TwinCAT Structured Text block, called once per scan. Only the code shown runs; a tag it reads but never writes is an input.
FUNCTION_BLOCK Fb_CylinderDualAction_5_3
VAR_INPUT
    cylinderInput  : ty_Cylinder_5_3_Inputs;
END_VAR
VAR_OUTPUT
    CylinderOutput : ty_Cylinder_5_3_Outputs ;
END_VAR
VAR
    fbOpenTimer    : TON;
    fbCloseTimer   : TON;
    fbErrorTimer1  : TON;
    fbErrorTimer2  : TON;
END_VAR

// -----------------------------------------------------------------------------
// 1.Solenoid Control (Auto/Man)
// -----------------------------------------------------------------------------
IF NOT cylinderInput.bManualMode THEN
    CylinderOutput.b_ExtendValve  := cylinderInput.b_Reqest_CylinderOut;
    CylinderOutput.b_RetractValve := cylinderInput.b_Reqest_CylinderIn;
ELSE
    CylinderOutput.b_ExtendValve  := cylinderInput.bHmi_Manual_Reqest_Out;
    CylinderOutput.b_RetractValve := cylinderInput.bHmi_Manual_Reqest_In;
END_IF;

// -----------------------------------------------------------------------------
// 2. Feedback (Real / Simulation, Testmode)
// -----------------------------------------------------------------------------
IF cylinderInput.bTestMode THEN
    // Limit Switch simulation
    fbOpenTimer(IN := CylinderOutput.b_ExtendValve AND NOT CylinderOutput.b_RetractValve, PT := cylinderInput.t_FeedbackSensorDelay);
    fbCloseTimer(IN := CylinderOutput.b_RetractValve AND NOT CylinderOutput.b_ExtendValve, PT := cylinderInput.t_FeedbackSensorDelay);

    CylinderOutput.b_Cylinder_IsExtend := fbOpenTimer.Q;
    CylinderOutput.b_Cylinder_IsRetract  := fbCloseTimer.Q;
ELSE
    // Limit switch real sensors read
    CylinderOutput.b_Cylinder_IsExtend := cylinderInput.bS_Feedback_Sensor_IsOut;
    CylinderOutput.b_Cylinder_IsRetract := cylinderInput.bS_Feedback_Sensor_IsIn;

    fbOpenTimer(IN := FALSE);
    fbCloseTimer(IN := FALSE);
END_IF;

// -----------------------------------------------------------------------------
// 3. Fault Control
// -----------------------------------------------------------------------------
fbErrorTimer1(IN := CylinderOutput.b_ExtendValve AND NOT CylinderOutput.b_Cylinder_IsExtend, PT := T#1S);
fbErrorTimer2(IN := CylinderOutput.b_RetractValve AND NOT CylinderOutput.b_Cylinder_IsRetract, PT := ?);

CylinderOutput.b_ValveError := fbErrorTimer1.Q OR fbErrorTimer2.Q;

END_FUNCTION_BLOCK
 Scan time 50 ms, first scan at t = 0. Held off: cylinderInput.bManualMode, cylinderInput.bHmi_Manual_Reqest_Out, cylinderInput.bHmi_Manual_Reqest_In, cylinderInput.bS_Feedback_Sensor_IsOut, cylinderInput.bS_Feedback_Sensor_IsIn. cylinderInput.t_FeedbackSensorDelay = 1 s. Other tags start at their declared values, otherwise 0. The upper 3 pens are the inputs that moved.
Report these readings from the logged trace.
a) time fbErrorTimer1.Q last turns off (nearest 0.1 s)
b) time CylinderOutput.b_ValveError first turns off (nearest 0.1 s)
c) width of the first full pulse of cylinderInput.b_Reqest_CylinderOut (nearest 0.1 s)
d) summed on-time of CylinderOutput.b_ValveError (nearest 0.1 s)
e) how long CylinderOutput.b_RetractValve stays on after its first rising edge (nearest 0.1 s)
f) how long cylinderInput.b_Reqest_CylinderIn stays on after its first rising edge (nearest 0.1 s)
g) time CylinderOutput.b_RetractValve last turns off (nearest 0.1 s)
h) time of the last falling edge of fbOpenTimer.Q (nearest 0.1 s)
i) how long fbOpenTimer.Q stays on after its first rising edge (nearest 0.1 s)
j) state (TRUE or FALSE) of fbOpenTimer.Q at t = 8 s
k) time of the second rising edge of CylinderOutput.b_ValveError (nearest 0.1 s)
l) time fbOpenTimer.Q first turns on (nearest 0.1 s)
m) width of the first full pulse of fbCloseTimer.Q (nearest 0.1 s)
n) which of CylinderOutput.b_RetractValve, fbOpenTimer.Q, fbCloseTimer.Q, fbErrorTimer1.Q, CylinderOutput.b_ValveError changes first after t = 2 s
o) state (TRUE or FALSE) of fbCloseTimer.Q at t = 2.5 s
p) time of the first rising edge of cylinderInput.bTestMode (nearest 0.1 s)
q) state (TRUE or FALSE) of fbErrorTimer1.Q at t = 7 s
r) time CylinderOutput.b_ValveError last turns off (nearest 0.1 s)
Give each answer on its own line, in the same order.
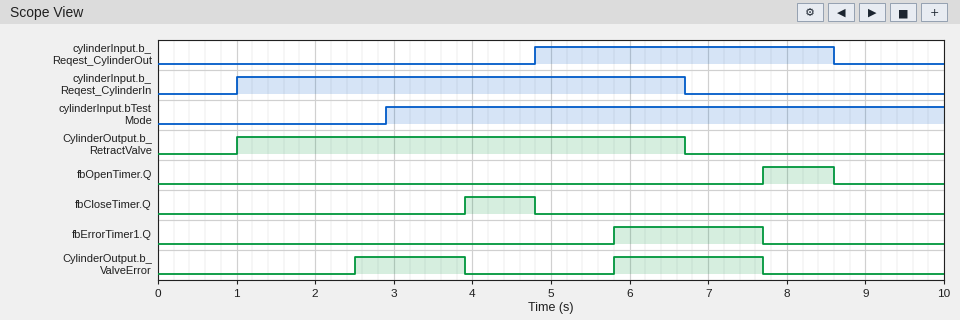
7.7 s
3.9 s
3.8 s
3.3 s
5.7 s
5.7 s
6.7 s
8.6 s
0.9 s
TRUE
5.8 s
7.7 s
0.9 s
CylinderOutput.b_ValveError
FALSE
2.9 s
TRUE
7.7 s
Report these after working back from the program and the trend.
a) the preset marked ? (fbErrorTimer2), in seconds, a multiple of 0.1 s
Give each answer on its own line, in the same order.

1.5 s
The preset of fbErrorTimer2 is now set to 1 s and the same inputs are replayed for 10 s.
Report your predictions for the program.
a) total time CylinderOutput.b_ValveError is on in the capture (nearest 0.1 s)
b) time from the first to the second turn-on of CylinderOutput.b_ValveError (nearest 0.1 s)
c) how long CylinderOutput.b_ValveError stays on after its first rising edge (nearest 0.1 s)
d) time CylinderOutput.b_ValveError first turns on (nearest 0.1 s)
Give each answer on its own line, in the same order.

3.8 s
3.8 s
1.9 s
2.0 s
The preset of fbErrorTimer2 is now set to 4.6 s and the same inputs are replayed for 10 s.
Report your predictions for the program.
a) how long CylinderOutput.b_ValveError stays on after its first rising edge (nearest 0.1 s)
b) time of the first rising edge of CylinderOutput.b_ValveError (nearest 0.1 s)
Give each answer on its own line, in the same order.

1.9 s
5.8 s
